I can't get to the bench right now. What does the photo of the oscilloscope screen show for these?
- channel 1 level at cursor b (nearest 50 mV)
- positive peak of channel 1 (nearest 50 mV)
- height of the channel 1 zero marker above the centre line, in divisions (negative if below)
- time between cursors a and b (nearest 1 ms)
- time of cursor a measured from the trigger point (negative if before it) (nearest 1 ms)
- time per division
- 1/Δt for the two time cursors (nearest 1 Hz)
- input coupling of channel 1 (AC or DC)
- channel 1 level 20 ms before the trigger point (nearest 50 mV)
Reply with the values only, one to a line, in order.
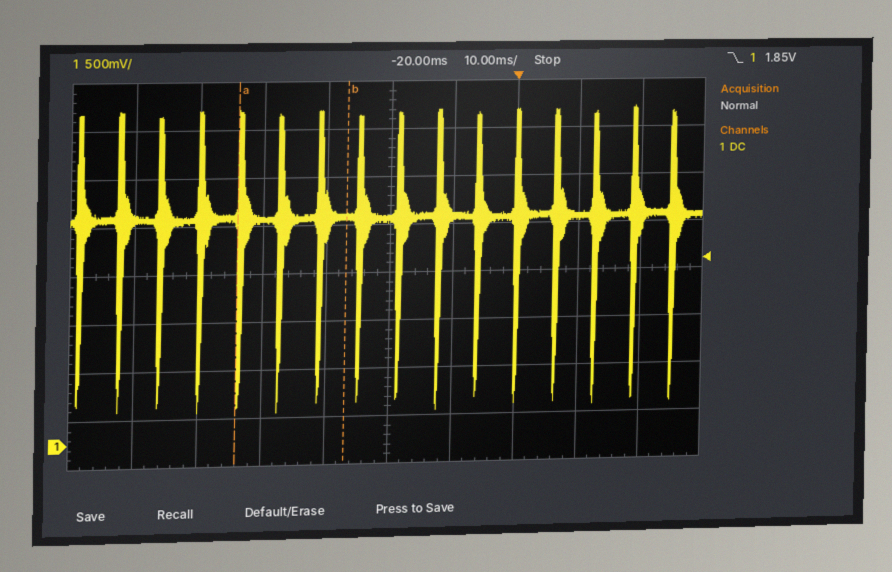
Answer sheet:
2.35 V
3.45 V
-3.5 div
17 ms
-44 ms
10 ms
59 Hz
DC
2.30 V
